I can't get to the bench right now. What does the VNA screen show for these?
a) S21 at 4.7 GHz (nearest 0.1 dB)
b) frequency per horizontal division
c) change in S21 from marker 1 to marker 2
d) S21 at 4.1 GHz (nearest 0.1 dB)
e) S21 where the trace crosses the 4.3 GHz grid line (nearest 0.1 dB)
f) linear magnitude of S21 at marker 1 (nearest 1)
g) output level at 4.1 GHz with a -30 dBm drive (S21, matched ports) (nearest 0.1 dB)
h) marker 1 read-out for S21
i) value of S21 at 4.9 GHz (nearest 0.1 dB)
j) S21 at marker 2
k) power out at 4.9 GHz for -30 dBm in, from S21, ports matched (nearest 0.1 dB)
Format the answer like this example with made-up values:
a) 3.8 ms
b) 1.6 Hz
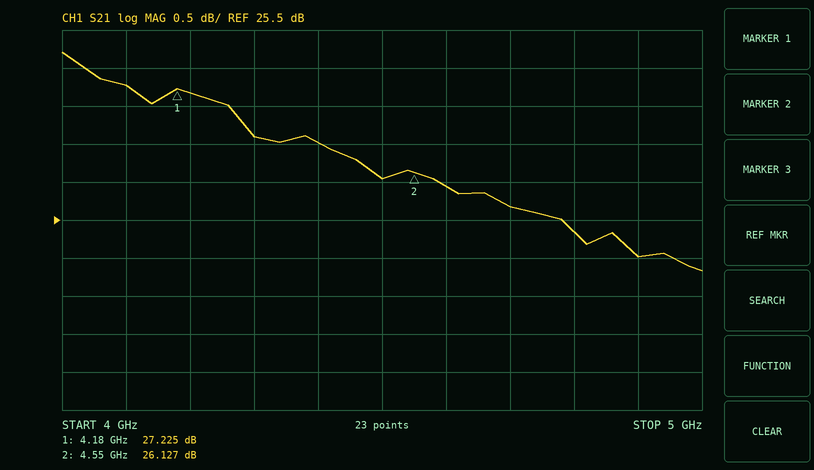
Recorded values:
a) 25.7 dB
b) 100 MHz
c) -1.098 dB
d) 27.3 dB
e) 26.6 dB
f) 23
g) -2.7 dBm
h) 27.225 dB
i) 25.0 dB
j) 26.127 dB
k) -5.0 dBm
